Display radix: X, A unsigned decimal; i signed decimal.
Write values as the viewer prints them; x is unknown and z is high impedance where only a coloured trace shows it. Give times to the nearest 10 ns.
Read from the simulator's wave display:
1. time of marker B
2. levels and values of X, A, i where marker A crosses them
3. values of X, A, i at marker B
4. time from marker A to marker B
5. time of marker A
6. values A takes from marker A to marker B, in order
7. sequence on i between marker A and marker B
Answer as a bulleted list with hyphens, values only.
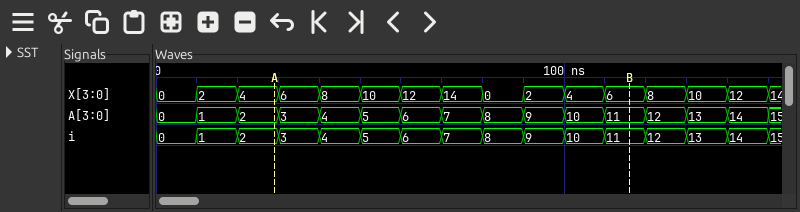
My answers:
- 120 ns
- X=4, A=2, i=2
- X=6, A=11, i=11
- 90 ns
- 30 ns
- 2, 3, 4, 5, 6, 7, 8, 9, 10, 11
- 2, 3, 4, 5, 6, 7, 8, 9, 10, 11
